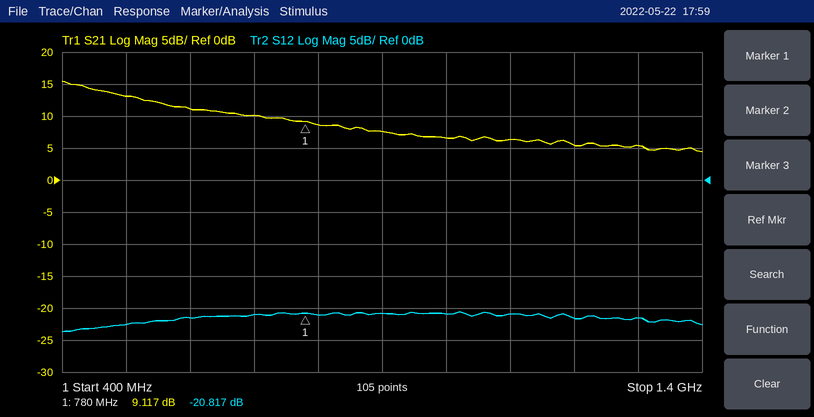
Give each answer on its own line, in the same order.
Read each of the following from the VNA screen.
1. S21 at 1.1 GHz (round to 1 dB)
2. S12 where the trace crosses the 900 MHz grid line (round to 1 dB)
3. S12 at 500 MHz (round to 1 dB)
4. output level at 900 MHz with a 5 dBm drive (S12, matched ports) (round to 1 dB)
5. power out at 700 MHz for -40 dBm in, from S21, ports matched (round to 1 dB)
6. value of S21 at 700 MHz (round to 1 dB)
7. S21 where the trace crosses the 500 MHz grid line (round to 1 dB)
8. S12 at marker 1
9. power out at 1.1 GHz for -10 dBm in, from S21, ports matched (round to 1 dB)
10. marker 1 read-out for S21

6 dB
-21 dB
-23 dB
-16 dBm
-30 dBm
10 dB
13 dB
-20.817 dB
-4 dBm
9.117 dB
